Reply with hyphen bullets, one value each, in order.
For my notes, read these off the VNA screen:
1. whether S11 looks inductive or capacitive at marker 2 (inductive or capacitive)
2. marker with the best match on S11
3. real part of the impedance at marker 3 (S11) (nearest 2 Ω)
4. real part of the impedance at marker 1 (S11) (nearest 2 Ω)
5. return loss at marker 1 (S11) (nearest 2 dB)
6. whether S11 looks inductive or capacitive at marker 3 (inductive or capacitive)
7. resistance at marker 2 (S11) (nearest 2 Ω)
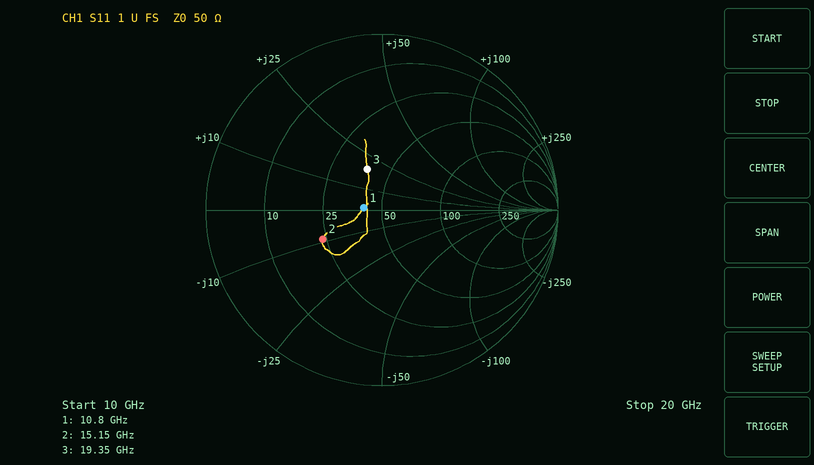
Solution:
- capacitive
- marker 1
- 38 Ω
- 40 Ω
- 20 dB
- inductive
- 24 Ω
